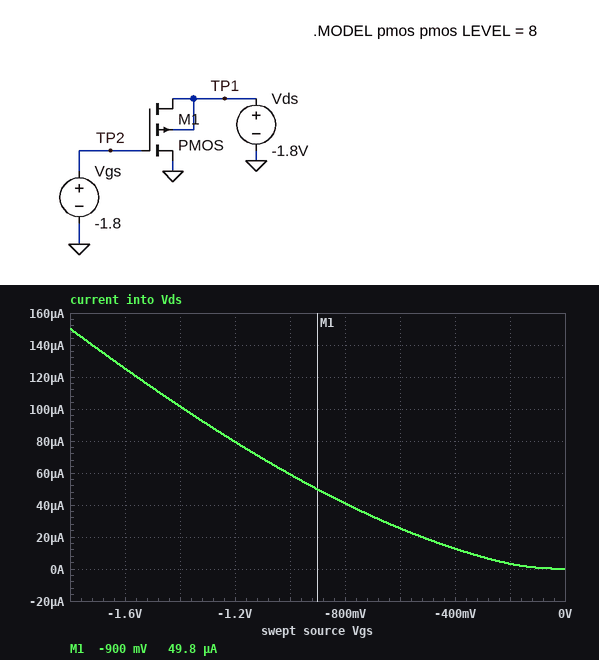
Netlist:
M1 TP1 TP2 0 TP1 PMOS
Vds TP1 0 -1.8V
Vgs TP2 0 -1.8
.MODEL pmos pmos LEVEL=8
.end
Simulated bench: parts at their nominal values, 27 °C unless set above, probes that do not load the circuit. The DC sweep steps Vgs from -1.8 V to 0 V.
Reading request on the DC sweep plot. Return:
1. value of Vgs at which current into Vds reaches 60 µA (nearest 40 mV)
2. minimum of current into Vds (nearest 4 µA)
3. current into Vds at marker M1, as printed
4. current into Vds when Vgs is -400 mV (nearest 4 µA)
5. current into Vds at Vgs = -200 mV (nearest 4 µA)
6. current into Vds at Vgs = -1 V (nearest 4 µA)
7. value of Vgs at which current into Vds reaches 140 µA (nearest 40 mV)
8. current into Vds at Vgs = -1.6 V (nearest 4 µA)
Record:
-1.00 V
0 A
49.8 µA
12 µA
4 µA
60 µA
-1.72 V
124 µA
